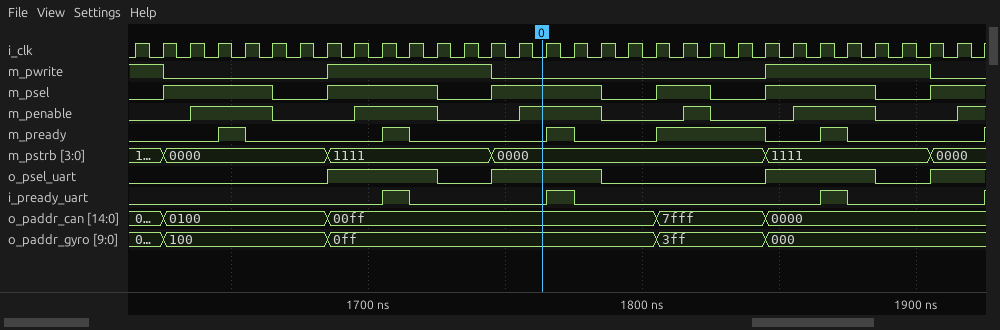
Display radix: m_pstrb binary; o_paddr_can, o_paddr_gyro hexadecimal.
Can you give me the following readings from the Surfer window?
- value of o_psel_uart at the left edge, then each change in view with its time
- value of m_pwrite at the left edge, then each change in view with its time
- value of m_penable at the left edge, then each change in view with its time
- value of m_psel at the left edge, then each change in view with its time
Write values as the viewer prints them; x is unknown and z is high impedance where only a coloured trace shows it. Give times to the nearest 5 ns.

0, 1 at 1685 ns, 0 at 1725 ns, 1 at 1745 ns, 0 at 1785 ns, 1 at 1845 ns, 0 at 1885 ns, 1 at 1905 ns
1, 0 at 1625 ns, 1 at 1685 ns, 0 at 1745 ns, 1 at 1845 ns, 0 at 1905 ns
0, 1 at 1635 ns, 0 at 1665 ns, 1 at 1695 ns, 0 at 1725 ns, 1 at 1755 ns, 0 at 1785 ns, 1 at 1815 ns, 0 at 1825 ns, 1 at 1855 ns, 0 at 1885 ns, 1 at 1915 ns
0, 1 at 1625 ns, 0 at 1665 ns, 1 at 1685 ns, 0 at 1725 ns, 1 at 1745 ns, 0 at 1785 ns, 1 at 1805 ns, 0 at 1825 ns, 1 at 1845 ns, 0 at 1885 ns, 1 at 1905 ns
